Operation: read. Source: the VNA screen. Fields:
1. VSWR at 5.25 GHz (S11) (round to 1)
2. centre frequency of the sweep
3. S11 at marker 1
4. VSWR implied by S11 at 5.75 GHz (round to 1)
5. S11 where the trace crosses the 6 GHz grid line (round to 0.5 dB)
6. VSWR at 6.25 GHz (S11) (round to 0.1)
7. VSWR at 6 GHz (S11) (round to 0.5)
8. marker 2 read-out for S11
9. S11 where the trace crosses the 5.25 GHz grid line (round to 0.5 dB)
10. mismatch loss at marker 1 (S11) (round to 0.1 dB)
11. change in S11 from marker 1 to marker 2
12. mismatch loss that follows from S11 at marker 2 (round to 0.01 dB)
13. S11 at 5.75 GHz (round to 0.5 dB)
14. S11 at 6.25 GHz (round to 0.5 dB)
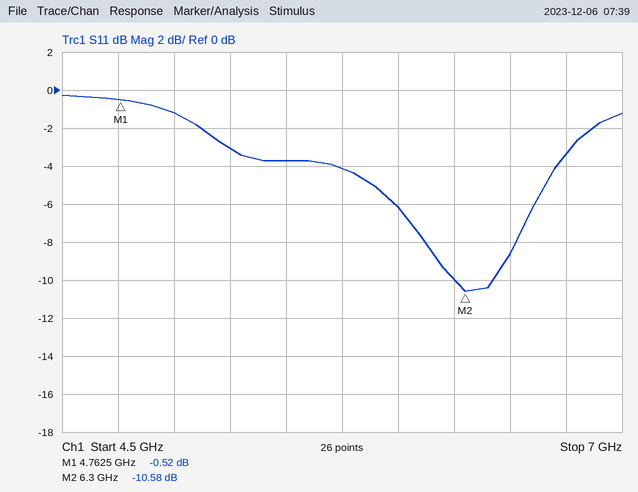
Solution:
6
5.75 GHz
-0.52 dB
4
-6.0 dB
1.9
3.0
-10.58 dB
-3.0 dB
9.5 dB
-10.06 dB
0.40 dB
-4.0 dB
-10.0 dB
